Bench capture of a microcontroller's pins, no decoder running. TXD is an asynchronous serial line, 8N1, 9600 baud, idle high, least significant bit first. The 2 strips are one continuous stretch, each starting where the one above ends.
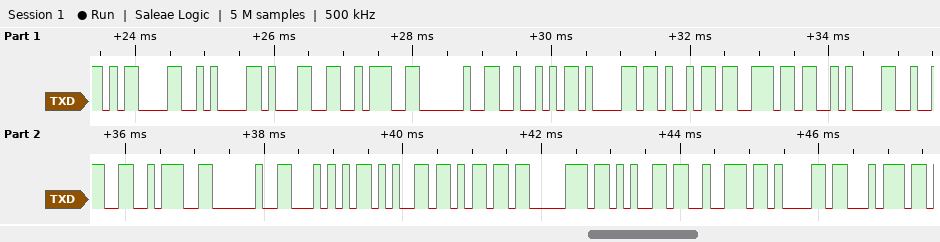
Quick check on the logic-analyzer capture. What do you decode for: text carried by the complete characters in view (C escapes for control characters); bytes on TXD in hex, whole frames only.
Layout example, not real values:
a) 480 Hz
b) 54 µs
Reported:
a) "\r\n1: Rain\n2: Temperat"
b) 0D 0A 31 3A 20 52 61 69 6E 0A 32 3A 20 54 65 6D 70 65 72 61 74
